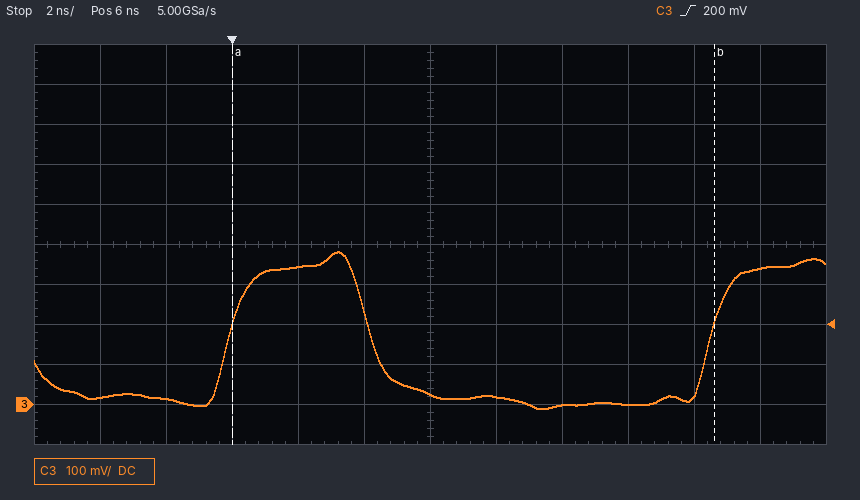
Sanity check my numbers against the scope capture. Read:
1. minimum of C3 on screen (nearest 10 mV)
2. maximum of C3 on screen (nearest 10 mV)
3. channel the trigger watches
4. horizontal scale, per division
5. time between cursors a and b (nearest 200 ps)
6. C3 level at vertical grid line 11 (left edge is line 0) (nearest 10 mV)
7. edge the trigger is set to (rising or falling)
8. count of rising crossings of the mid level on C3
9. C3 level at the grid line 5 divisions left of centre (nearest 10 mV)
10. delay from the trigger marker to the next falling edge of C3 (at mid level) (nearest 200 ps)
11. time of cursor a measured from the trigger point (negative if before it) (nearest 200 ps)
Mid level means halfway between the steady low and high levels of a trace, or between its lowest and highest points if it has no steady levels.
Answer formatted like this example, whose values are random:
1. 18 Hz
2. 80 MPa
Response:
1. -10 mV
2. 380 mV
3. C3
4. 2 ns
5. 14.6 ns
6. 340 mV
7. rising
8. 2
9. 20 mV
10. 4.2 ns
11. 0.0 ns
